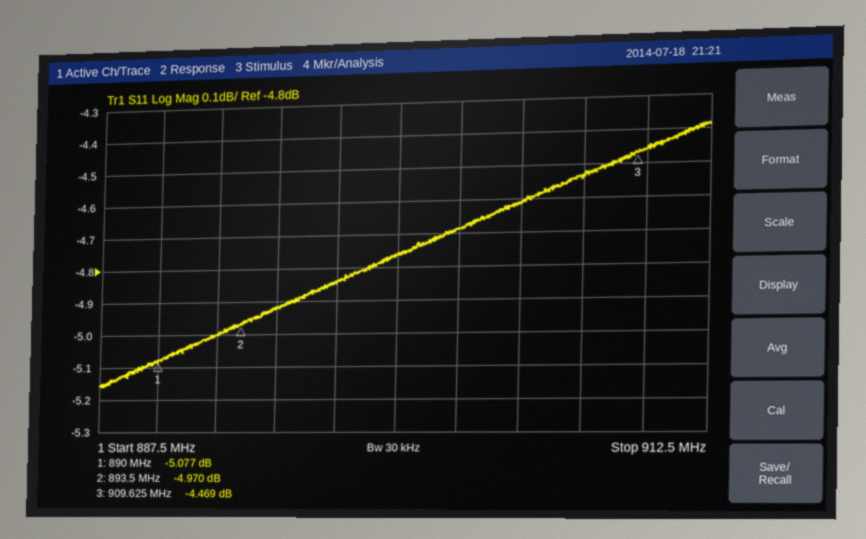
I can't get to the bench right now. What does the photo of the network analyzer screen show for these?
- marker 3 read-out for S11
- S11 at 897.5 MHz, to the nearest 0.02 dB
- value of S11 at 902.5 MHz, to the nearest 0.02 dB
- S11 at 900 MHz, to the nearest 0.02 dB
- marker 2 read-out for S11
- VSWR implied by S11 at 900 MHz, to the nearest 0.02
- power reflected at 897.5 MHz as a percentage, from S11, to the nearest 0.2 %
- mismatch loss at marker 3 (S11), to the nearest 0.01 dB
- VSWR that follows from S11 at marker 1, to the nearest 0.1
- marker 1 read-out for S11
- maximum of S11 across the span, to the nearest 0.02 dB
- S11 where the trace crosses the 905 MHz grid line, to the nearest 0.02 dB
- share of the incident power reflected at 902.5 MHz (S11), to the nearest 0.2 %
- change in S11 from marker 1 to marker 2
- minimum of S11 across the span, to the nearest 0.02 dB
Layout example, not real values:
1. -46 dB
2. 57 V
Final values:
1. -4.469 dB
2. -4.84 dB
3. -4.68 dB
4. -4.76 dB
5. -4.970 dB
6. 3.74
7. 32.8 %
8. 1.92 dB
9. 3.5
10. -5.077 dB
11. -4.38 dB
12. -4.62 dB
13. 34.0 %
14. 0.107 dB
15. -5.16 dB
